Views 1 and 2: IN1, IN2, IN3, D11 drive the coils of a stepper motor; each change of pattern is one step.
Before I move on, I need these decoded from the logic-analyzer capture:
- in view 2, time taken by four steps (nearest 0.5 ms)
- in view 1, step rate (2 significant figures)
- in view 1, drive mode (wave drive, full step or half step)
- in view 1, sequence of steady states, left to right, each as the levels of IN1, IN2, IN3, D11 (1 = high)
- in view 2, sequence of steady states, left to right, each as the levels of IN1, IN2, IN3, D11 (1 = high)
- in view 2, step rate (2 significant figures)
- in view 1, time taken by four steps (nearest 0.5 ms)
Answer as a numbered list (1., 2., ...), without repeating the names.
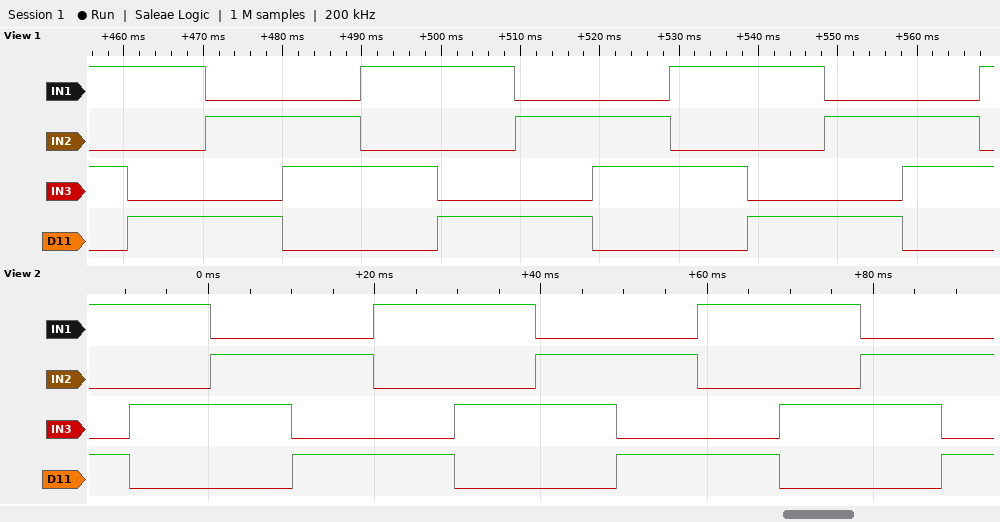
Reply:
1. 39.0 ms
2. 100 steps/s
3. full step
4. 1010 1001 0101 0110 1010 1001 0101 0110 1010 1001 0101 0110 1010
5. 1001 1010 0110 0101 1001 1010 0110 0101 1001 1010 0110 0101
6. 100 steps/s
7. 39.0 ms
